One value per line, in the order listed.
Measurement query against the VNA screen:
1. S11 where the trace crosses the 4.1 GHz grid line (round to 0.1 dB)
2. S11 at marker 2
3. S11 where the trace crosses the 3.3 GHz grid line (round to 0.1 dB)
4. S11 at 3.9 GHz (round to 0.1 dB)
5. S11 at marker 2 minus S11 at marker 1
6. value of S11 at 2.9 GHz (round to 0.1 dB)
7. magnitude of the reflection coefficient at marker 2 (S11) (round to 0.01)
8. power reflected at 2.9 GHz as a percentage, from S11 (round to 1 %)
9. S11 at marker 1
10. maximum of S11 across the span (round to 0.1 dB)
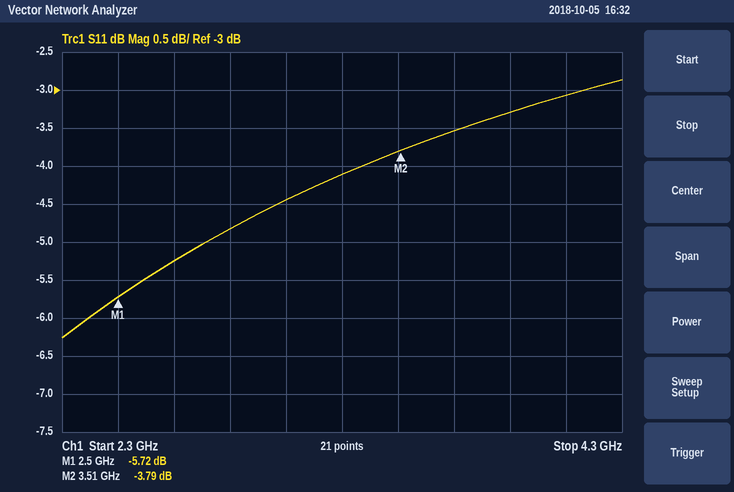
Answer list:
-3.1 dB
-3.79 dB
-4.1 dB
-3.3 dB
1.93 dB
-4.8 dB
0.65
33 %
-5.72 dB
-2.9 dB
